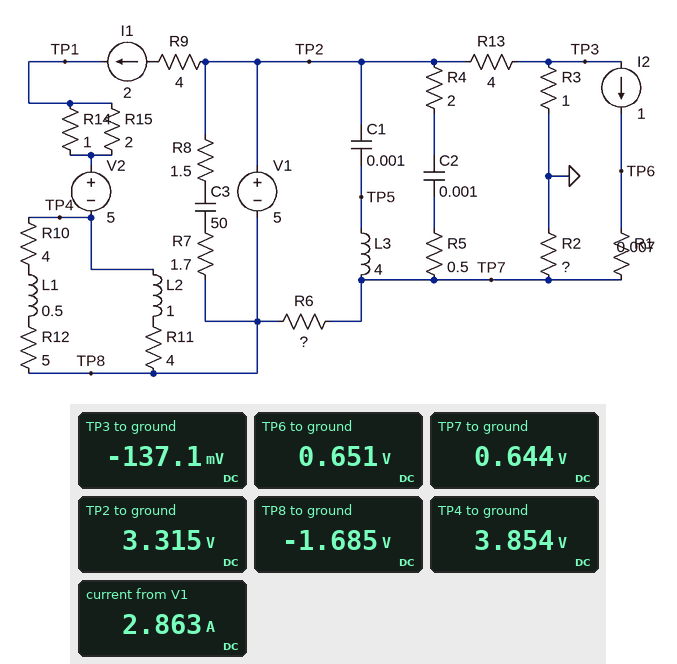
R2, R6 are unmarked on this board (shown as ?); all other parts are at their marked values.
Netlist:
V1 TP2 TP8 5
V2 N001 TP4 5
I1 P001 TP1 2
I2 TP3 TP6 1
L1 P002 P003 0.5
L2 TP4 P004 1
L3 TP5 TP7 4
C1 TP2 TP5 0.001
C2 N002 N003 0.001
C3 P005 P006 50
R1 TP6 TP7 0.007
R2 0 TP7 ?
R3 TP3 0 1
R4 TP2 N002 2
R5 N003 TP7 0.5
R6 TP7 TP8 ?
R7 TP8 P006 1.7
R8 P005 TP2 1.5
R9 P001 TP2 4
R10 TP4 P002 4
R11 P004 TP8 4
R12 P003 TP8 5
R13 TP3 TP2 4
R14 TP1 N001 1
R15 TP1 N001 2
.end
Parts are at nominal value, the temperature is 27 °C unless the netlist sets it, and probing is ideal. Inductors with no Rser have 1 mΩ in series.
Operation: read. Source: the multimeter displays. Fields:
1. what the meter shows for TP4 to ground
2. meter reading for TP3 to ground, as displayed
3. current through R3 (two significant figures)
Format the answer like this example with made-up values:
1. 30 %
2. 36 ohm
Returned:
1. 3.854 V
2. -137.1 mV
3. 140 mA
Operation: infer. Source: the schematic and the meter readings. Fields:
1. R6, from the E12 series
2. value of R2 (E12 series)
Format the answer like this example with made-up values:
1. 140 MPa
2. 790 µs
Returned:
1. 2.7 Ω
2. 4.7 Ω
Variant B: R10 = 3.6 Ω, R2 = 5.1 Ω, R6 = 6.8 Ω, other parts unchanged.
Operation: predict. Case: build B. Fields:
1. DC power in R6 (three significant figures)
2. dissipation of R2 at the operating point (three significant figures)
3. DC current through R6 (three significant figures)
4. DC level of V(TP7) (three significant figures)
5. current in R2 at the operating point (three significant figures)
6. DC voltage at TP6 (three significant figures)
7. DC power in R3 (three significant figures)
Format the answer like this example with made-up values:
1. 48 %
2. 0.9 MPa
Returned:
1. 2.93 W
2. 601 mW
3. 657 mA
4. 1.75 V
5. 343 mA
6. 1.76 V
7. 118 mW
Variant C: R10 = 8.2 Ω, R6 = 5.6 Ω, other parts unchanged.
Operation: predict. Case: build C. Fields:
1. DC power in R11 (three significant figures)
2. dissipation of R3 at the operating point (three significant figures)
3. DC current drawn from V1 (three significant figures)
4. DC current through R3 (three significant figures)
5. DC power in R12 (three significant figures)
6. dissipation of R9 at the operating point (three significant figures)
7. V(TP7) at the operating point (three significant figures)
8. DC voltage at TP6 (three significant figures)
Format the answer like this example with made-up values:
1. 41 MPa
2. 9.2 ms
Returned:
1. 9.42 W
2. 90.4 mW
3. 2.70 A
4. 301 mA
5. 1.08 W
6. 16.0 W
7. 1.41 V
8. 1.42 V
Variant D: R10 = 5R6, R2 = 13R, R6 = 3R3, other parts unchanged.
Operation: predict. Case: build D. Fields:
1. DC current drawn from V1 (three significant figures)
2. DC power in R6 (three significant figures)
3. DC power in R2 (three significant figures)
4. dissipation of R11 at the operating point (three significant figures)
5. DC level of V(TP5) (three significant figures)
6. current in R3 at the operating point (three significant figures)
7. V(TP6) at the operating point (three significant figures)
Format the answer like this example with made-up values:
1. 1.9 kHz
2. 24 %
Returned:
1. 2.89 A
2. 2.63 W
3. 152 mW
4. 8.43 W
5. 1.40 V
6. 108 mA
7. 1.41 V
